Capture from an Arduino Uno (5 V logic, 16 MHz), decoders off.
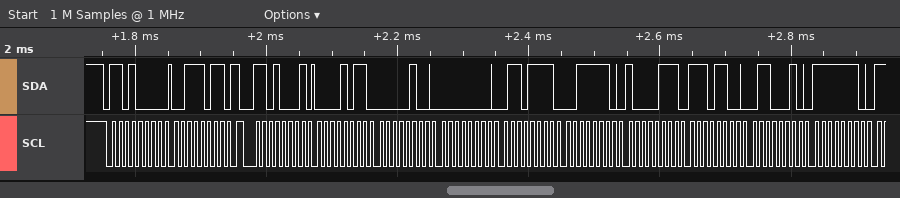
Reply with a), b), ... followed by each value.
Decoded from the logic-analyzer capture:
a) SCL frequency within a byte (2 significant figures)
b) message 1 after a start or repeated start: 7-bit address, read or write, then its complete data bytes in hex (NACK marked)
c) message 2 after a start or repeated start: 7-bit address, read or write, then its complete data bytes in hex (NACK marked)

a) 100 kHz
b) 0x68 write: 3B
c) 0x68 read: 0B 04 00 6F 3E 87 EC 62 FE
